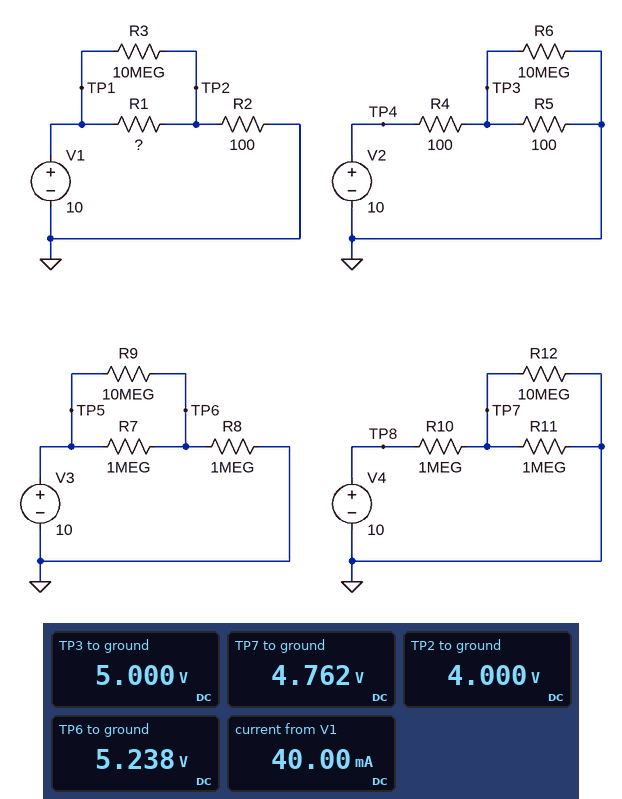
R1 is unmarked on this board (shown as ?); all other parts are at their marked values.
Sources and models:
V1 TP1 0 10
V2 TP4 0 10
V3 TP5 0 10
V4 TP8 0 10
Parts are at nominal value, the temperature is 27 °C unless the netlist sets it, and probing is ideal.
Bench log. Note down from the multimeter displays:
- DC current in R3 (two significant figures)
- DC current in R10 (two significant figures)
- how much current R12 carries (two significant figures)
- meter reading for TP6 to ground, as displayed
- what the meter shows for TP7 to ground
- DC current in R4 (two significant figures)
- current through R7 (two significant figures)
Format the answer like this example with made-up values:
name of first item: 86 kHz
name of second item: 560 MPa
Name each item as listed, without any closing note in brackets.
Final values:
DC current in R3: 600 nA
DC current in R10: 5.2 µA
how much current R12 carries: 480 nA
meter reading for TP6 to ground, as displayed: 5.238 V
what the meter shows for TP7 to ground: 4.762 V
DC current in R4: 50 mA
current through R7: 4.8 µA
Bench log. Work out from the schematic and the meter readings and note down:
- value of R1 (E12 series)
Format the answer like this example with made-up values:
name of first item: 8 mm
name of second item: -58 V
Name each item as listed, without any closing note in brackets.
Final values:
value of R1: 150 Ω
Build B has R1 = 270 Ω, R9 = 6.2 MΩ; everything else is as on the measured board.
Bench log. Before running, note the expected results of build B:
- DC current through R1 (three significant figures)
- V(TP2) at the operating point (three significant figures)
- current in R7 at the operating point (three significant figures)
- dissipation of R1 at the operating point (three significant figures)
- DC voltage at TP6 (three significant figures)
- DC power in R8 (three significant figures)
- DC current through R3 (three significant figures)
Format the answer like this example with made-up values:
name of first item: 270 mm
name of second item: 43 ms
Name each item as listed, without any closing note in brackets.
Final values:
DC current through R1: 27.0 mA
V(TP2) at the operating point: 2.70 V
current in R7 at the operating point: 4.63 µA
dissipation of R1 at the operating point: 197 mW
DC voltage at TP6: 5.37 V
DC power in R8: 28.9 µW
DC current through R3: 730 nA
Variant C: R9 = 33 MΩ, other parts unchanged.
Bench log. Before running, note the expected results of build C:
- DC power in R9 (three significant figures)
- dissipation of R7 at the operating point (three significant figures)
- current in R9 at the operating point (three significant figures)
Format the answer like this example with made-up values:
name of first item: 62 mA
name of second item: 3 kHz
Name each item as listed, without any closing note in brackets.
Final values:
DC power in R9: 735 nW
dissipation of R7 at the operating point: 24.3 µW
current in R9 at the operating point: 149 nA
